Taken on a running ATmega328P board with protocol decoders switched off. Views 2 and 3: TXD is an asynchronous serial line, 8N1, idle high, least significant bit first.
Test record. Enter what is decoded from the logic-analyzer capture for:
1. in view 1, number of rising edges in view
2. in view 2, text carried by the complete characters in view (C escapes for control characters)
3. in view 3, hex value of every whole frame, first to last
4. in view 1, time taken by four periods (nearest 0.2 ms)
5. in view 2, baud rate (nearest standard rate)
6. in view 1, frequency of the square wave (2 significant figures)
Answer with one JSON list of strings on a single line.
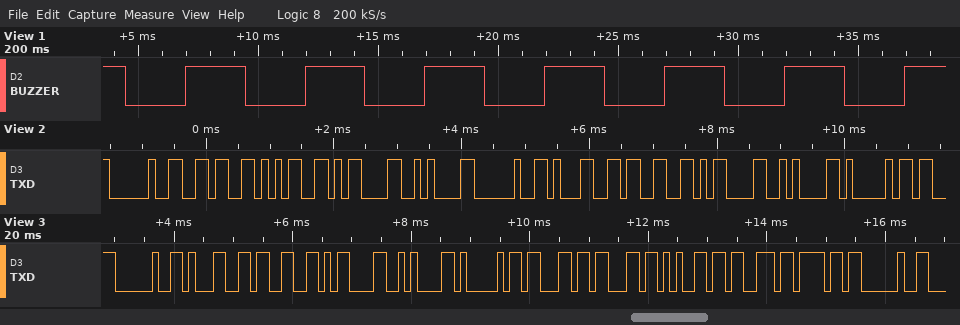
["7", "\" 65\\r\\n 13\\r\\nA\"", "20 31 33 0D 0A 41 63 63 65 73 6F 20", "20.0 ms", "9600 baud", "200 Hz"]
